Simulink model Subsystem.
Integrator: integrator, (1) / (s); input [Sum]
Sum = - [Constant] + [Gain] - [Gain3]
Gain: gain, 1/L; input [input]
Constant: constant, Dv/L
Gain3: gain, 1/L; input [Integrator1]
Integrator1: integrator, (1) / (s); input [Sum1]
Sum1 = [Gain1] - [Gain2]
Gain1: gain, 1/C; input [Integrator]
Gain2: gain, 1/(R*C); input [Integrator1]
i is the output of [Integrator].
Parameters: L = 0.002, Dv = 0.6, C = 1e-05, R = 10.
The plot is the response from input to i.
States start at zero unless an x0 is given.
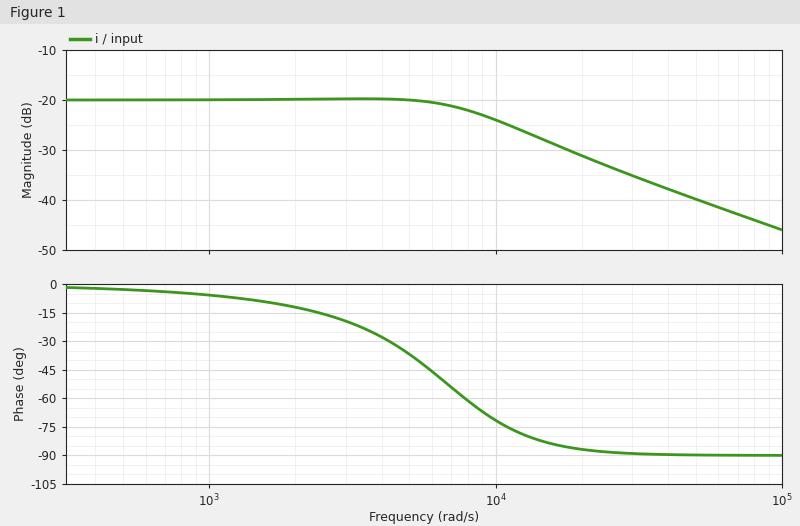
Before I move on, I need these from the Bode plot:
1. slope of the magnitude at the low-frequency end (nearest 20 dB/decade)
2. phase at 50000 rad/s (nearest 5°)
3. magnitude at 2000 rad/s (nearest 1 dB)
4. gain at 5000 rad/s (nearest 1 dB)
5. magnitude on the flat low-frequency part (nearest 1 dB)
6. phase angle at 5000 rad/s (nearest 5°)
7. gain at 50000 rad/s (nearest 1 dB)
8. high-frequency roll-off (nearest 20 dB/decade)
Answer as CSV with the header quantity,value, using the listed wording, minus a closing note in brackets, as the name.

quantity,value
slope of the magnitude at the low-frequency end,0 dB/decade
phase at 50000 rad/s,-90°
magnitude at 2000 rad/s,-20 dB
gain at 5000 rad/s,-20 dB
magnitude on the flat low-frequency part,-20 dB
phase angle at 5000 rad/s,-35°
gain at 50000 rad/s,-40 dB
high-frequency roll-off,-20 dB/decade
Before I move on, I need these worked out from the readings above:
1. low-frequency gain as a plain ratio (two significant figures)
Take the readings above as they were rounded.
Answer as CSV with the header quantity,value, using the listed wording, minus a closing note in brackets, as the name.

quantity,value
low-frequency gain as a plain ratio,0.10
